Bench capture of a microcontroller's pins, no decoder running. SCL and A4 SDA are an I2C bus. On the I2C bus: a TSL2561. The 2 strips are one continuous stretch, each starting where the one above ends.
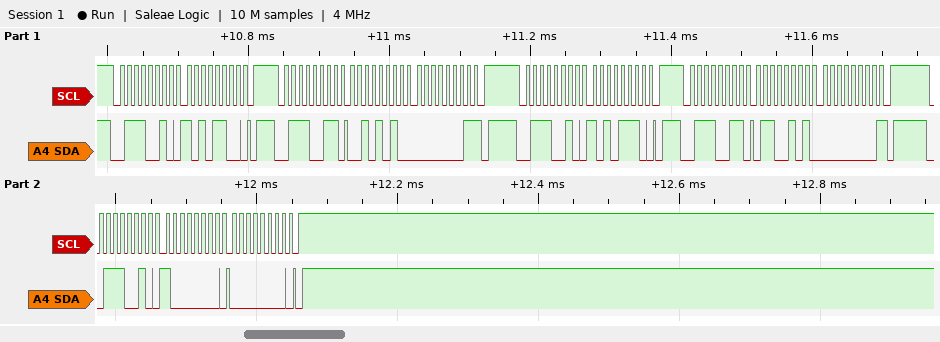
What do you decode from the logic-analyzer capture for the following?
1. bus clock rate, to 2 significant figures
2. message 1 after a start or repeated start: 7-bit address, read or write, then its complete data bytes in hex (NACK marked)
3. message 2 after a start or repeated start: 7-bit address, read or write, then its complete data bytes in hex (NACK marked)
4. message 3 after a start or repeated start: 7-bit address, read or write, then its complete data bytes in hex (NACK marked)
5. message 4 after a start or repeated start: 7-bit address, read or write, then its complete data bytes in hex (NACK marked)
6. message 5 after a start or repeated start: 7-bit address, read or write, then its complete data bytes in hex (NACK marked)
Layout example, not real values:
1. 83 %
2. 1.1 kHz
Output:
1. 100 kHz
2. 0x39 write: AC
3. 0x39 read: 2A 01 NACK
4. 0x39 write: AE
5. 0x39 read: 65 00 NACK
6. 0x39 write: 80 00
